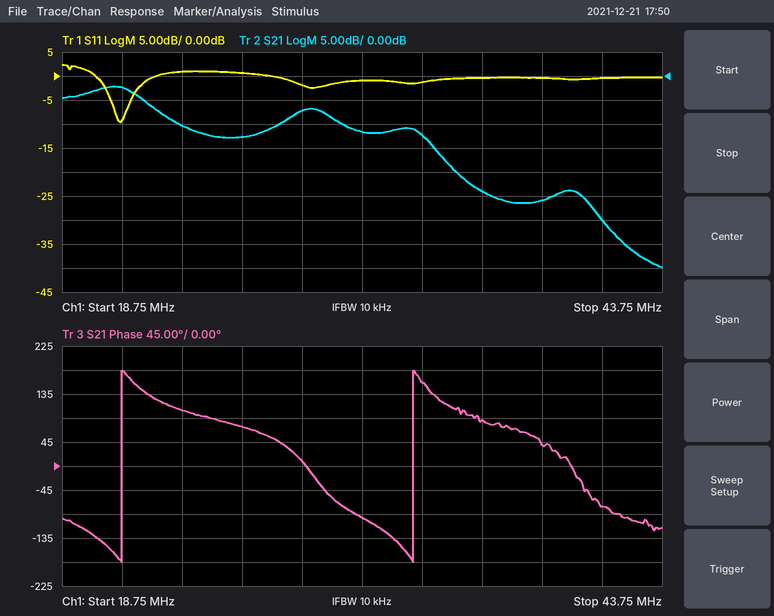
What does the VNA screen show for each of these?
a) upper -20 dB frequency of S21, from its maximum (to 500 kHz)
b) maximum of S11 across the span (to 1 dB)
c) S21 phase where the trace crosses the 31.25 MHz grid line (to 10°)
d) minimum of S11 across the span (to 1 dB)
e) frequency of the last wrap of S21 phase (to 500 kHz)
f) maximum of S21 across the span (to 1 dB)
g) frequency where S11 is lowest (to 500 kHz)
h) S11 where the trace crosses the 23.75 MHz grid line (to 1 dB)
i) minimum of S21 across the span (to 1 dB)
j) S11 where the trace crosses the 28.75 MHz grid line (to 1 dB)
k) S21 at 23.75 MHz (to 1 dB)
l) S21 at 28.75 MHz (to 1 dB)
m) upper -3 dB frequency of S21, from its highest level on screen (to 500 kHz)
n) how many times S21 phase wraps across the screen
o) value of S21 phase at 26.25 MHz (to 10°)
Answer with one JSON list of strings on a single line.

["35.5 MHz", "2 dB", "-100°", "-10 dB", "33.5 MHz", "-2 dB", "21.0 MHz", "1 dB", "-40 dB", "-2 dB", "-10 dB", "-7 dB", "22.0 MHz", "2", "70°"]
